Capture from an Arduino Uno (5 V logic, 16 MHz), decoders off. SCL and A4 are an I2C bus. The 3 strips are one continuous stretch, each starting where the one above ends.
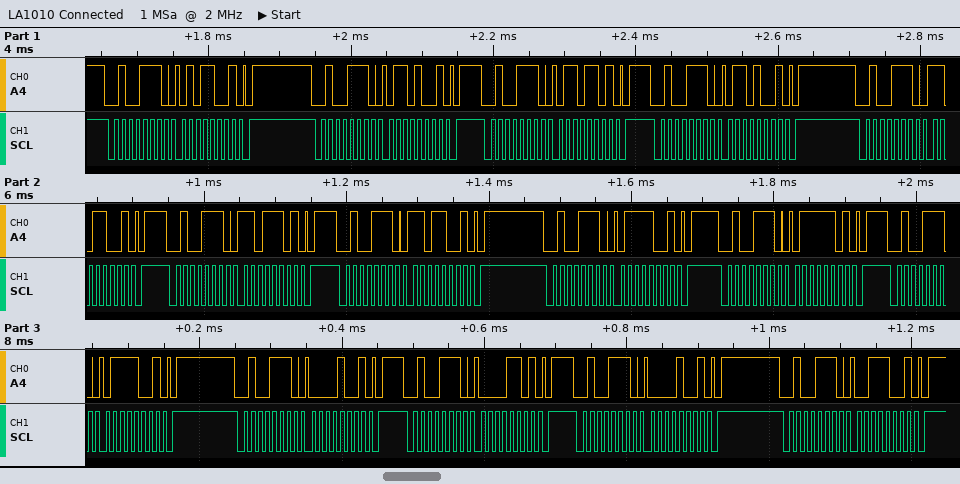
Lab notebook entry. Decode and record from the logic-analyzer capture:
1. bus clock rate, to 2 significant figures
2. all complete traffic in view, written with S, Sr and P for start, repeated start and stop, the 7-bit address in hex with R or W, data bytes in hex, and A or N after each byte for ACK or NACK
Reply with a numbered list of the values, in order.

1. 100 kHz
2. S 27W A 59 A P S 27W A 69 A P S 27W A 6D A P S 27W A 69 A P S 27W A D9 A P S 27W A DD A P S 27W A D9 A P S 27W A 79 A P S 27W A 7D A P S 27W A 79 A P S 27W A 09 A P S 27W A 0D A P S 27W A 09 A P S 27W A 39 A P
